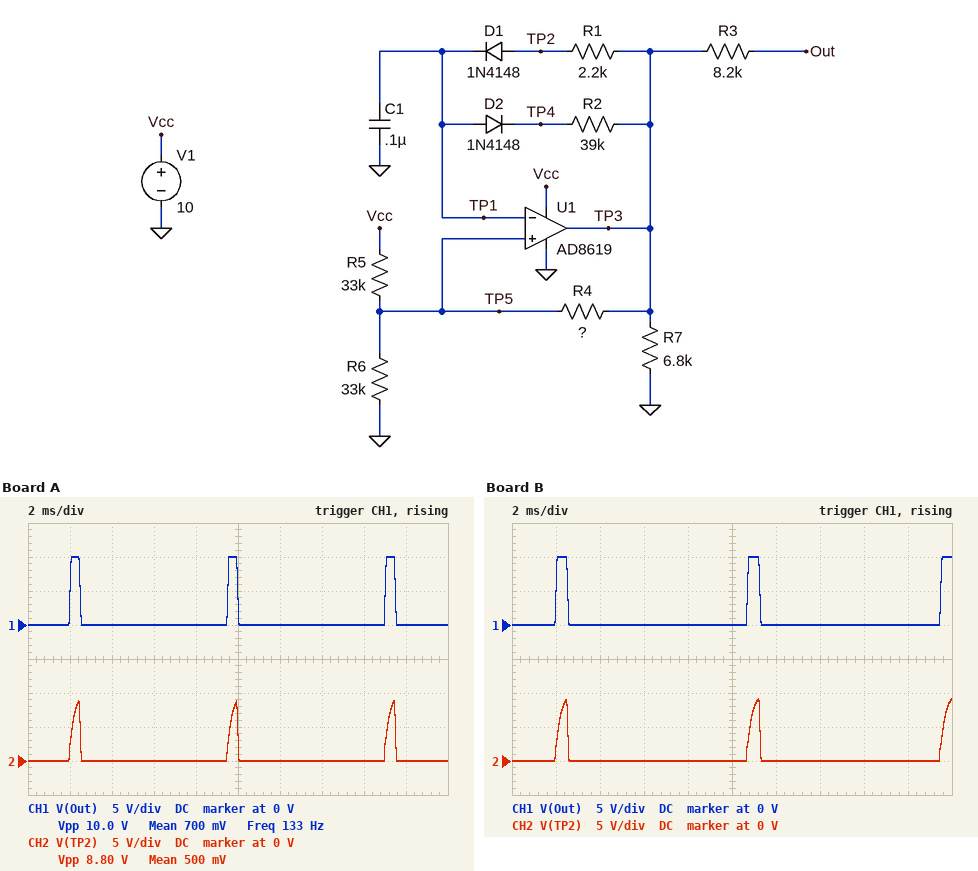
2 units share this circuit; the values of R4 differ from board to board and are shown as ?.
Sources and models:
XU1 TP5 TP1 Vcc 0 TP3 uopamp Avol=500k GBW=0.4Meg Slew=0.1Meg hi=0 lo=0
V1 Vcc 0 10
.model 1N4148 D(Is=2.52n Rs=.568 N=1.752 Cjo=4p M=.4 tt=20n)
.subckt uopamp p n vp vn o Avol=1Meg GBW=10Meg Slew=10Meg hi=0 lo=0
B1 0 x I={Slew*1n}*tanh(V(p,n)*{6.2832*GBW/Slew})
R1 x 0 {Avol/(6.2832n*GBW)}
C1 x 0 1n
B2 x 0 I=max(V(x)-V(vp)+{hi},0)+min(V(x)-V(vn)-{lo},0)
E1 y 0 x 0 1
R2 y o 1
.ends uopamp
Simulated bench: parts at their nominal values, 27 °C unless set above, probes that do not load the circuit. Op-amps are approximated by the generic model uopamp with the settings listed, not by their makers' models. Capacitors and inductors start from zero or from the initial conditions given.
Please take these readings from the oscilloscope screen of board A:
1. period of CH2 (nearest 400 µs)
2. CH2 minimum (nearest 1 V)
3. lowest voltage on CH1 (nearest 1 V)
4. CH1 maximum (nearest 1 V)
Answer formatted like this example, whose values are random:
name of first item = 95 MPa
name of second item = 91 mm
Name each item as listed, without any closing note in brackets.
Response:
period of CH2 = 7.6 ms
CH2 minimum = 0 V
lowest voltage on CH1 = 0 V
CH1 maximum = 10 V
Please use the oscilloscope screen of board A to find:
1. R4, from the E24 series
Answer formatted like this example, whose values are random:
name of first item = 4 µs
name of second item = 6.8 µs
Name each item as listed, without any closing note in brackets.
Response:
R4, from the E24 series = 9.1 kΩ
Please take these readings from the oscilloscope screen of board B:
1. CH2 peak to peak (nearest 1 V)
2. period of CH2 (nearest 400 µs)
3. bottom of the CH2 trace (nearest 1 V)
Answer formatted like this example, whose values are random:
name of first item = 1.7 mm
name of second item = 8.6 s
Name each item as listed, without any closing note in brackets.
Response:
CH2 peak to peak = 9 V
period of CH2 = 8.8 ms
bottom of the CH2 trace = 0 V
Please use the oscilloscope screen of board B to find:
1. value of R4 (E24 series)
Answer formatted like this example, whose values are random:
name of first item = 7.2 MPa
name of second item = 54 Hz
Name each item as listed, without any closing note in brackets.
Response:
value of R4 = 6.8 kΩ
